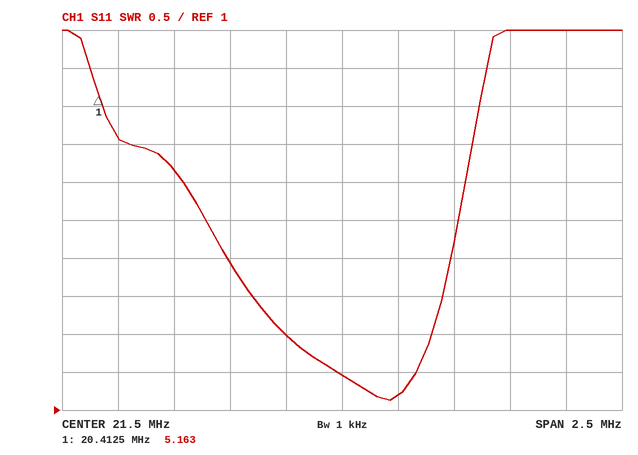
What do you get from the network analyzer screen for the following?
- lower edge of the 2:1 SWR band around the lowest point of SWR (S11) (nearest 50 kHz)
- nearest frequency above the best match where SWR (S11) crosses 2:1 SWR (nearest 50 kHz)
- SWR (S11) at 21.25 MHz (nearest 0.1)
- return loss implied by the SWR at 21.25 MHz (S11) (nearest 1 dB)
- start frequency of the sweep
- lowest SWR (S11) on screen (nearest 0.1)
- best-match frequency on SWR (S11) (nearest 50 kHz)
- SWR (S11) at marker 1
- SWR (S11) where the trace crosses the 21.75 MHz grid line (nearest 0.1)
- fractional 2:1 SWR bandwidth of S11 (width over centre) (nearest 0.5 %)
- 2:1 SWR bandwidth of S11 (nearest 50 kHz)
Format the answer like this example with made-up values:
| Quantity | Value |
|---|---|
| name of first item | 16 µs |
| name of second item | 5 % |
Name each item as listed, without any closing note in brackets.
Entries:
| Quantity | Value |
|---|---|
| lower edge of the 2:1 SWR band around the lowest point of SWR (S11) | 21.25 MHz |
| nearest frequency above the best match where SWR (S11) crosses 2:1 SWR | 21.90 MHz |
| SWR (S11) at 21.25 MHz | 2.0 |
| return loss implied by the SWR at 21.25 MHz (S11) | 10 dB |
| start frequency of the sweep | 20.25 MHz |
| lowest SWR (S11) on screen | 1.1 |
| best-match frequency on SWR (S11) | 21.70 MHz |
| SWR (S11) at marker 1 | 5.163 |
| SWR (S11) where the trace crosses the 21.75 MHz grid line | 1.2 |
| fractional 2:1 SWR bandwidth of S11 (width over centre) | 3.0 % |
| 2:1 SWR bandwidth of S11 | 650 kHz |
